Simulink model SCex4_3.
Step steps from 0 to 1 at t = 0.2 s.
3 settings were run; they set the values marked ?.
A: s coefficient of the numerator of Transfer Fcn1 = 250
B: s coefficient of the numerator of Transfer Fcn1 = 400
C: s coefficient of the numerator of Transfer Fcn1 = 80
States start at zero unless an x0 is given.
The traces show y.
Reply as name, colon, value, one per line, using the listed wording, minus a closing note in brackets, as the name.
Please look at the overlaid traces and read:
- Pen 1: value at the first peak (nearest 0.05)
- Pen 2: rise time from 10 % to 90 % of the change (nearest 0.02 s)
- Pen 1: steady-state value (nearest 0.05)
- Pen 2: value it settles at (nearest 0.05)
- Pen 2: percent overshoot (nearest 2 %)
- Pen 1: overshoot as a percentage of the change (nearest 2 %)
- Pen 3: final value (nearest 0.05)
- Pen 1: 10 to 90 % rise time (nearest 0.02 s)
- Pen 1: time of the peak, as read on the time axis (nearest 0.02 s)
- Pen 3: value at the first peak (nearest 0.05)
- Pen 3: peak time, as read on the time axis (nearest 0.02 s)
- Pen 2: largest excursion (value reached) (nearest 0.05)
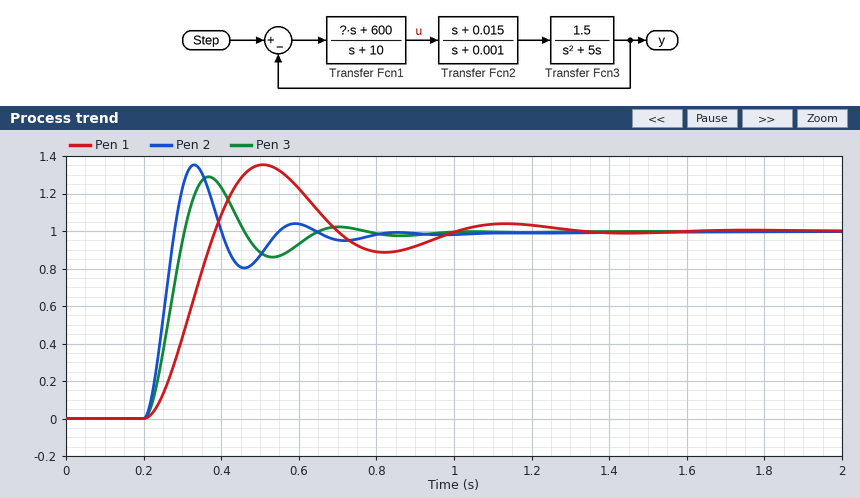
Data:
Pen 1: value at the first peak: 1.35
Pen 2: rise time from 10 % to 90 % of the change: 0.06 s
Pen 1: steady-state value: 1.00
Pen 2: value it settles at: 1.00
Pen 2: percent overshoot: 36 %
Pen 1: overshoot as a percentage of the change: 36 %
Pen 3: final value: 1.00
Pen 1: 10 to 90 % rise time: 0.12 s
Pen 1: time of the peak, as read on the time axis: 0.50 s
Pen 3: value at the first peak: 1.30
Pen 3: peak time, as read on the time axis: 0.36 s
Pen 2: largest excursion (value reached): 1.35
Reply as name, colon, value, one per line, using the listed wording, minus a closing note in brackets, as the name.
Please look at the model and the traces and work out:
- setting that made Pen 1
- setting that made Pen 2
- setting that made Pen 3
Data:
setting that made Pen 1: C
setting that made Pen 2: B
setting that made Pen 3: A
